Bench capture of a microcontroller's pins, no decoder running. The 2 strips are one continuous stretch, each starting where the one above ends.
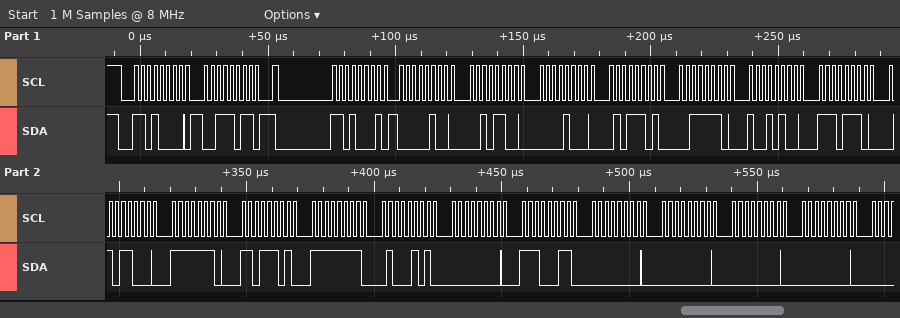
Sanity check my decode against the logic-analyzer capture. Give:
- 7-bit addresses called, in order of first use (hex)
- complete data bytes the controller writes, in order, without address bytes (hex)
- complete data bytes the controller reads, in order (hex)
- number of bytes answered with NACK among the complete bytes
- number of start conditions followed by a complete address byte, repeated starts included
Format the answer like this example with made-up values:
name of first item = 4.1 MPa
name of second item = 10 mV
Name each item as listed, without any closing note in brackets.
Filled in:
7-bit addresses called, in order of first use = 0x68
complete data bytes the controller writes, in order, without address bytes = 3B
complete data bytes the controller reads, in order = 04 2C 08 5D 3E 94 EE 58 FE DD FF 45 00 E3 00 00 00 00
number of bytes answered with NACK among the complete bytes = 0
number of start conditions followed by a complete address byte, repeated starts included = 2
